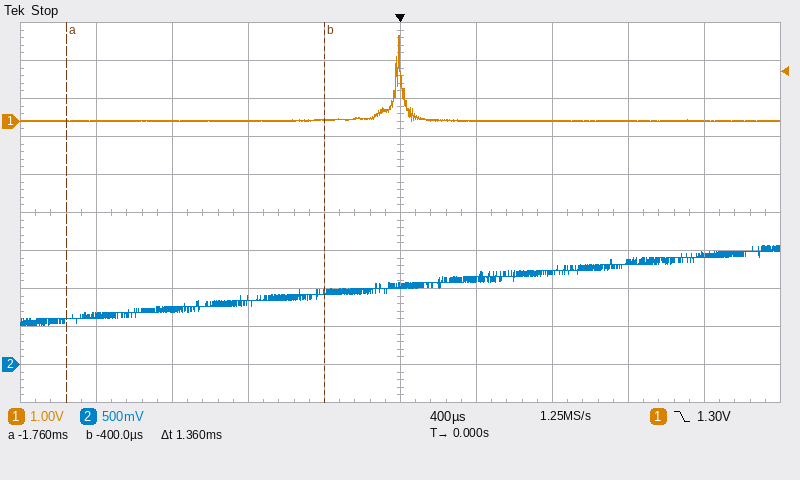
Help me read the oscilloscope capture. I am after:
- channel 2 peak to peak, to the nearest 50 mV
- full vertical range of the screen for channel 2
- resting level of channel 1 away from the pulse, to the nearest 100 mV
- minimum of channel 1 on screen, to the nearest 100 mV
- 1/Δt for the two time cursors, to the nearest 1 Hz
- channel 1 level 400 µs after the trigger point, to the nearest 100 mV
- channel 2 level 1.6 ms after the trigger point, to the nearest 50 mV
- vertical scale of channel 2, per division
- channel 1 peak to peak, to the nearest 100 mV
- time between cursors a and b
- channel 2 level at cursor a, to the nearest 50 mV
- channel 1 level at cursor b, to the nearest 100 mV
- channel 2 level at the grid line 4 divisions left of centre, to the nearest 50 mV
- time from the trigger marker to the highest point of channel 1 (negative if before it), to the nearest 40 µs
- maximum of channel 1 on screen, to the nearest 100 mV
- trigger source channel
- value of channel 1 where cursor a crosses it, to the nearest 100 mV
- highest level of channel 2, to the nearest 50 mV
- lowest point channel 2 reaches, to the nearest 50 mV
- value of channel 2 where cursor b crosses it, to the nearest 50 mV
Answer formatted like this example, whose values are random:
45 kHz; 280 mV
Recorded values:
1.05 V; 5 V; 0.0 V; 0.0 V; 735 Hz; 0.0 V; 1.45 V; 500 mV; 2.3 V; 1.36 ms; 550 mV; 0.0 V; 650 mV; 0 µs; 2.3 V; channel 1; 0.0 V; 1.55 V; 500 mV; 950 mV
